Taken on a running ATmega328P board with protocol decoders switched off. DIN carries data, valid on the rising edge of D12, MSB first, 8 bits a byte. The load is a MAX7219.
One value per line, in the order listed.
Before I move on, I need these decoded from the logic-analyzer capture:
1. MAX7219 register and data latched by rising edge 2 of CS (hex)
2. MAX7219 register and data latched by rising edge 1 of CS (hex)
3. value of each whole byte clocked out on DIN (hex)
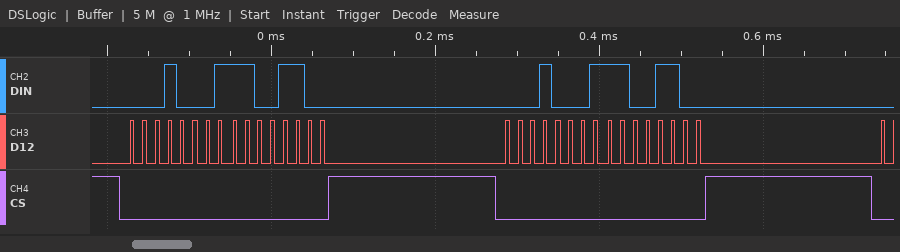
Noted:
register 0x1, data 0xCC
register 0x1, data 0xCC
11 CC 11 CC
